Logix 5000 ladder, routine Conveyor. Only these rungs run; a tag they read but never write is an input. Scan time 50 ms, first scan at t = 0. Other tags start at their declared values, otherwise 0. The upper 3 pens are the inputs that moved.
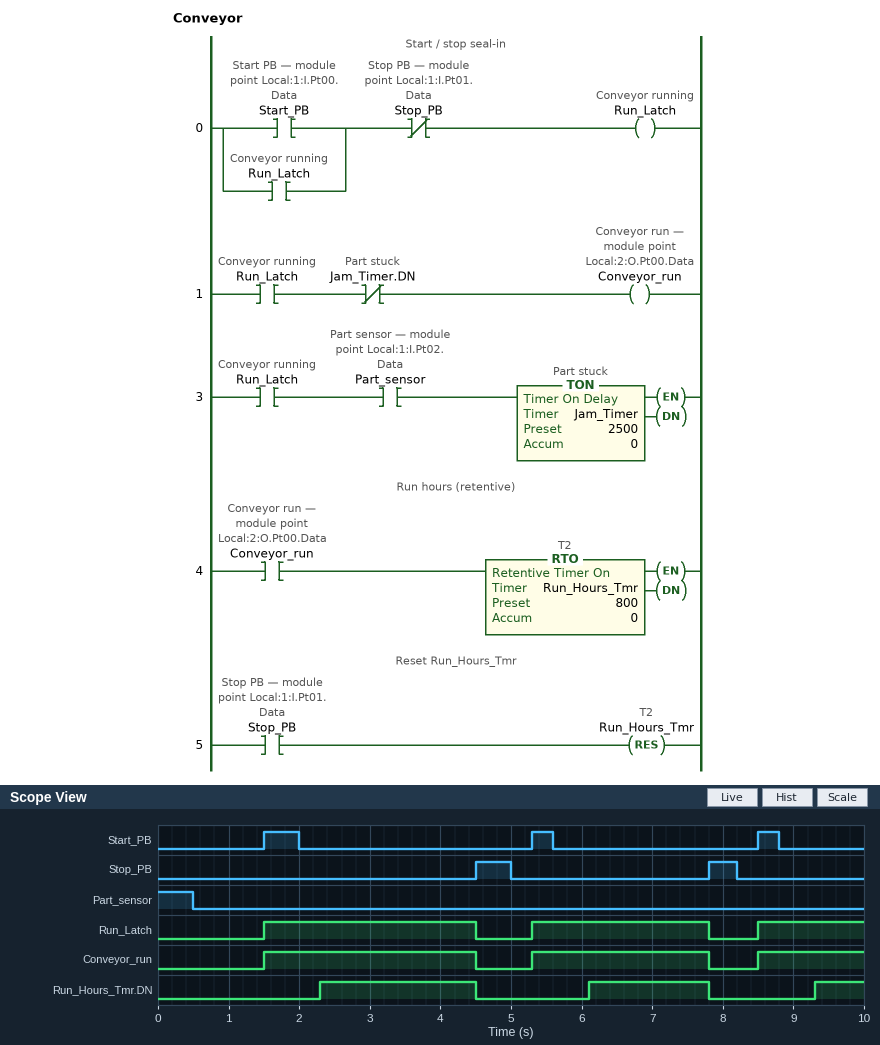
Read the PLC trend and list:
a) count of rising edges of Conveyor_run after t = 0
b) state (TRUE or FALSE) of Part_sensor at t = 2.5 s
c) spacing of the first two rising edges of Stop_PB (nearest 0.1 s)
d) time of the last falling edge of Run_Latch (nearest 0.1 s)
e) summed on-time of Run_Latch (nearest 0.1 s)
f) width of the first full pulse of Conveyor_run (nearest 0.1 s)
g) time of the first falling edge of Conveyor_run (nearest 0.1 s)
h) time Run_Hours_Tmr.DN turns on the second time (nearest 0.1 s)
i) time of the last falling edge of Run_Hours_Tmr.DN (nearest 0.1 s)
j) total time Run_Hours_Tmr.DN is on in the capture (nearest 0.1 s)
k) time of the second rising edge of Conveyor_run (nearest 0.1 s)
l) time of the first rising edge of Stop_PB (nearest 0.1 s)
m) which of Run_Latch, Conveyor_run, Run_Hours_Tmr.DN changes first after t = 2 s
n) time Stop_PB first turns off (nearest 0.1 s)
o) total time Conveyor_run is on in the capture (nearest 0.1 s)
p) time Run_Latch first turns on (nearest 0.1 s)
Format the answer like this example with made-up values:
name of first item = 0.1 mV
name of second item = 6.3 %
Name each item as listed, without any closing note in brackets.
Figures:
count of rising edges of Conveyor_run after t = 0 = 3
state (TRUE or FALSE) of Part_sensor at t = 2.5 s = FALSE
spacing of the first two rising edges of Stop_PB = 3.3 s
time of the last falling edge of Run_Latch = 7.8 s
summed on-time of Run_Latch = 7.0 s
width of the first full pulse of Conveyor_run = 3.0 s
time of the first falling edge of Conveyor_run = 4.5 s
time Run_Hours_Tmr.DN turns on the second time = 6.1 s
time of the last falling edge of Run_Hours_Tmr.DN = 7.8 s
total time Run_Hours_Tmr.DN is on in the capture = 4.6 s
time of the second rising edge of Conveyor_run = 5.3 s
time of the first rising edge of Stop_PB = 4.5 s
which of Run_Latch, Conveyor_run, Run_Hours_Tmr.DN changes first after t = 2 s = Run_Hours_Tmr.DN
time Stop_PB first turns off = 5.0 s
total time Conveyor_run is on in the capture = 7.0 s
time Run_Latch first turns on = 1.5 s
